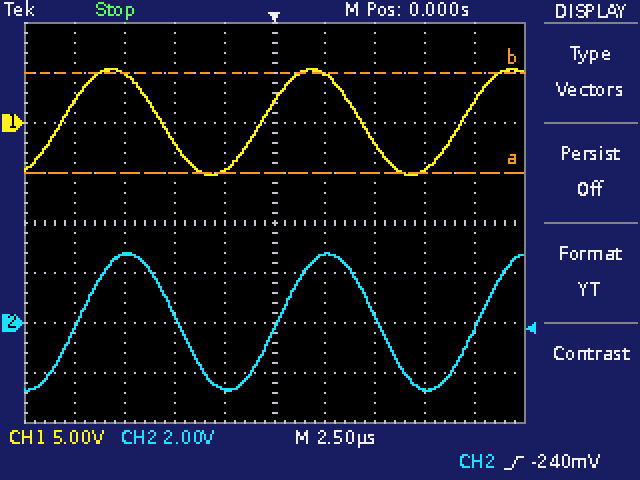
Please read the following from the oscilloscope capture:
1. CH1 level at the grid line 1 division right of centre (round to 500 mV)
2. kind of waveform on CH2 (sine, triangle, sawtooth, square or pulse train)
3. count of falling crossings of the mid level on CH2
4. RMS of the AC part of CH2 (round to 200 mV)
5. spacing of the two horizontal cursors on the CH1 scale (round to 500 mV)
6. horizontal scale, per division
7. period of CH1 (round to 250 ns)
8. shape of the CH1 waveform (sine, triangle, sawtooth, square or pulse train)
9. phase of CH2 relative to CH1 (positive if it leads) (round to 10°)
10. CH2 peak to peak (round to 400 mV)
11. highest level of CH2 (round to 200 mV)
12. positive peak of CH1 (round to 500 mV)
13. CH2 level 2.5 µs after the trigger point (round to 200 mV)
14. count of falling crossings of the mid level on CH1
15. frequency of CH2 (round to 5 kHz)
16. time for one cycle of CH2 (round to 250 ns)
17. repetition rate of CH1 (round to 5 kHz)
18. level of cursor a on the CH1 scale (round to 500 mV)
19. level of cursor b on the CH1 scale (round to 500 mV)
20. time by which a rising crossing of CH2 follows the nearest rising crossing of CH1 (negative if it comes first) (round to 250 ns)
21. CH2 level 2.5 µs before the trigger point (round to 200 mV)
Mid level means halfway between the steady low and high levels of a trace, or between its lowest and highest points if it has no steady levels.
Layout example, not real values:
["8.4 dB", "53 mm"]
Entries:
["5.0 V", "sine", "2", "2.0 V", "10.0 V", "2.5 µs", "10.00 µs", "sine", "-30°", "5.6 V", "2.8 V", "5.5 V", "2.8 V", "2", "100 kHz", "10.00 µs", "100 kHz", "-5.0 V", "5.0 V", "+750 ns", "-2.6 V"]
